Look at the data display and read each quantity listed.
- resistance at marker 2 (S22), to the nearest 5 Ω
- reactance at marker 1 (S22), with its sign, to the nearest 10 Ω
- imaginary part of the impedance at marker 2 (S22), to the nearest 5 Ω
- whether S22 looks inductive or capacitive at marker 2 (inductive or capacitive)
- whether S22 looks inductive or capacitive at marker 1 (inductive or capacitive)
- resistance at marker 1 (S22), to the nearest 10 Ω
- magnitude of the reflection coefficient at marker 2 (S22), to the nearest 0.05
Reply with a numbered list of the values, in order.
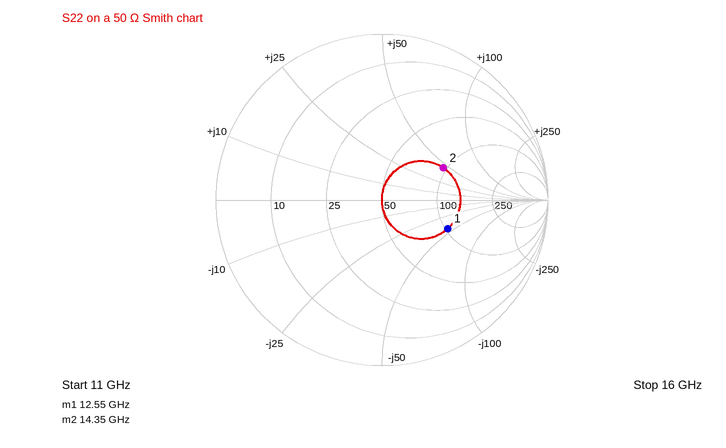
1. 95 Ω
2. -40 Ω
3. +45 Ω
4. inductive
5. capacitive
6. 100 Ω
7. 0.40
